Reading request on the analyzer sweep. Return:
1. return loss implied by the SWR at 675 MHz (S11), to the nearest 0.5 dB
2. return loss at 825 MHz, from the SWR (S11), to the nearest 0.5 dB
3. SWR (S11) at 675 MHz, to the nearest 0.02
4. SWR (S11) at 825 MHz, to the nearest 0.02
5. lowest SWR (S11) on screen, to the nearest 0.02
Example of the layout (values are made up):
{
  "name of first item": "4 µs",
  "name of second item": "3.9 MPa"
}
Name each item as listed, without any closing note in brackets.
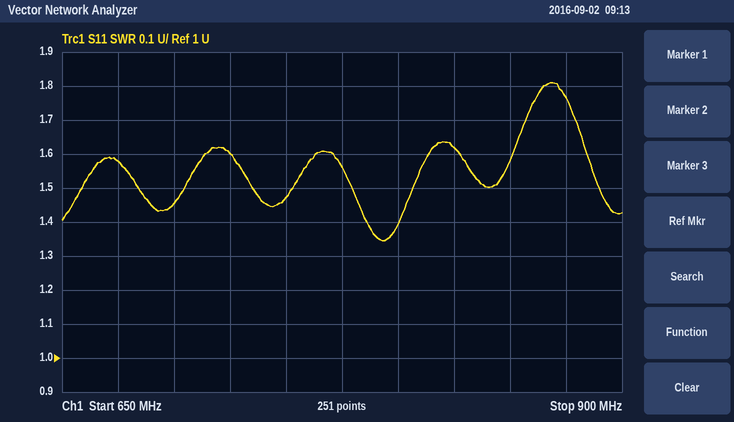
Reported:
{
  "return loss implied by the SWR at 675 MHz (S11), to the nearest 0.5 dB": "13.0 dB",
  "return loss at 825 MHz, from the SWR (S11), to the nearest 0.5 dB": "12.5 dB",
  "SWR (S11) at 675 MHz, to the nearest 0.02": "1.58",
  "SWR (S11) at 825 MHz, to the nearest 0.02": "1.62",
  "lowest SWR (S11) on screen, to the nearest 0.02": "1.34"
}
